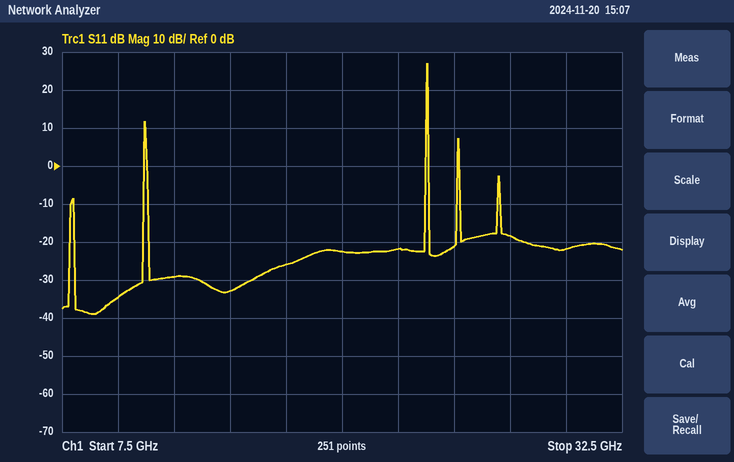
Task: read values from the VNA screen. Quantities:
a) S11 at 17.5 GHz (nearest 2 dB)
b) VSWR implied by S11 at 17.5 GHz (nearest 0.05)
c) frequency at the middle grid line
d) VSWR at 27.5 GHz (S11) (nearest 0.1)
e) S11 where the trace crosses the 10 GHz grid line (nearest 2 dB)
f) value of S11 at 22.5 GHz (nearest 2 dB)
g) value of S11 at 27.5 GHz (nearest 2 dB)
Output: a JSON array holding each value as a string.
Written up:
["-26 dB", "1.10", "20 GHz", "1.3", "-34 dB", "-22 dB", "-18 dB"]
